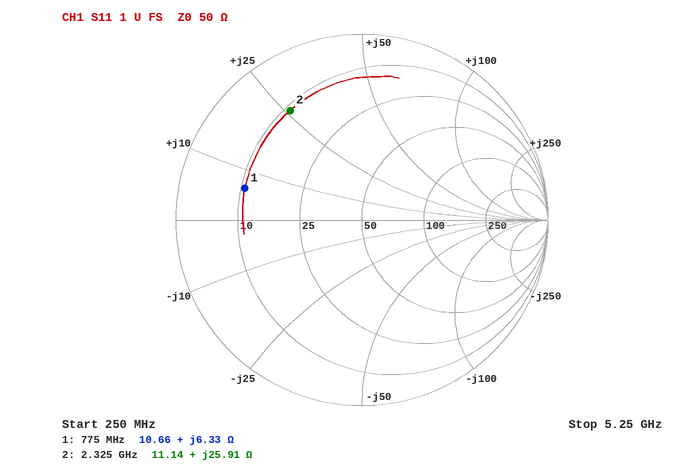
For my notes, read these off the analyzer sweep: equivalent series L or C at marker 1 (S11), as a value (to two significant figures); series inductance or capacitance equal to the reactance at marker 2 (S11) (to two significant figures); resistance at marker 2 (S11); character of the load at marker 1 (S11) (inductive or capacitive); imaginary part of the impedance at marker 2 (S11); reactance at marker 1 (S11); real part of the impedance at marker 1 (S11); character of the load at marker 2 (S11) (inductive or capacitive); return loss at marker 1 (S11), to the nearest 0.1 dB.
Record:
1.3 nH
1.8 nH
11.14 Ω
inductive
+25.91 Ω
+6.33 Ω
10.66 Ω
inductive
3.7 dB
